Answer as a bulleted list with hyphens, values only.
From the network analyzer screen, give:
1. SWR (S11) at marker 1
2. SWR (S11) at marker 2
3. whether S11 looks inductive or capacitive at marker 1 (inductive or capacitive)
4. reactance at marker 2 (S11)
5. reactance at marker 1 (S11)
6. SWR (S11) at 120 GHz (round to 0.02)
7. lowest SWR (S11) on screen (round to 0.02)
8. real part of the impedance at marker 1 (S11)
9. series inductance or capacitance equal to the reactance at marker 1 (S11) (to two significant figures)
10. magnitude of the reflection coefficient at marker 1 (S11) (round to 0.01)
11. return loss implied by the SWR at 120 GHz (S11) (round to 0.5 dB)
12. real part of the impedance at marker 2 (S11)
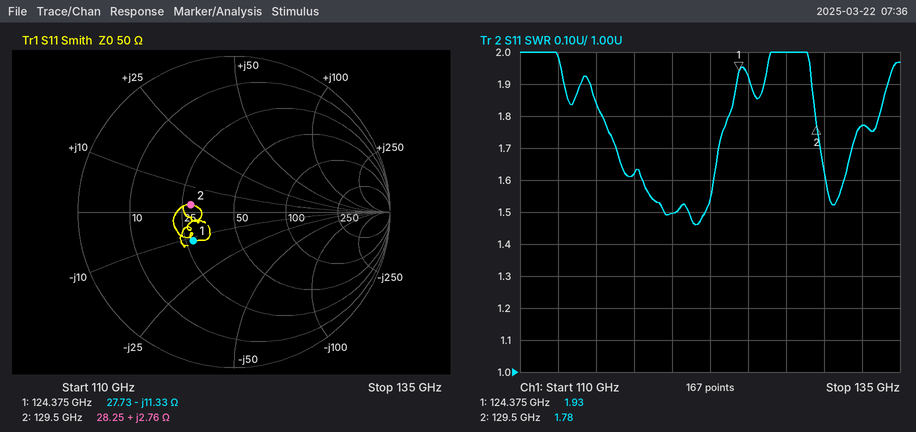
- 1.93
- 1.78
- capacitive
- +2.76 Ω
- -11.33 Ω
- 1.50
- 1.46
- 27.73 Ω
- 110 fF
- 0.32
- 14.0 dB
- 28.25 Ω
